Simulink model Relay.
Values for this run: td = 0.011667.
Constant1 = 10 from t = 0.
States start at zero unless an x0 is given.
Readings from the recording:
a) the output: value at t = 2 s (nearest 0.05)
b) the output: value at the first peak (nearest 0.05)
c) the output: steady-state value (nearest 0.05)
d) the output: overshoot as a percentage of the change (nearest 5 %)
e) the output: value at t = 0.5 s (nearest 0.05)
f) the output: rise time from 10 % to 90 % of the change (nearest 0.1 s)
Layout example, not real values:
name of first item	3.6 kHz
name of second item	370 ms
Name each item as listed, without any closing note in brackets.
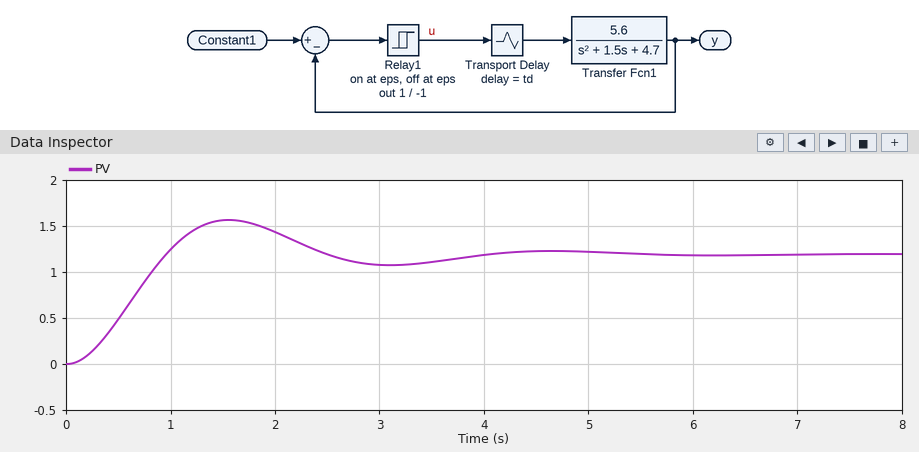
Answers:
the output: value at t = 2 s	1.45
the output: value at the first peak	1.55
the output: steady-state value	1.20
the output: overshoot as a percentage of the change	30 %
the output: value at t = 0.5 s	0.50
the output: rise time from 10 % to 90 % of the change	0.6 s
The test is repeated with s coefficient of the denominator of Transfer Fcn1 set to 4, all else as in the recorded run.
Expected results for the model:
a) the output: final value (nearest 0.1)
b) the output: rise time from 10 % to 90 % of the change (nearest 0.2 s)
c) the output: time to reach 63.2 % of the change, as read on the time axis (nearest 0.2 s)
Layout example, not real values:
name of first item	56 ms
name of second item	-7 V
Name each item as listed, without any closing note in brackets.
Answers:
the output: final value	1.2
the output: rise time from 10 % to 90 % of the change	1.4 s
the output: time to reach 63.2 % of the change, as read on the time axis	1.0 s
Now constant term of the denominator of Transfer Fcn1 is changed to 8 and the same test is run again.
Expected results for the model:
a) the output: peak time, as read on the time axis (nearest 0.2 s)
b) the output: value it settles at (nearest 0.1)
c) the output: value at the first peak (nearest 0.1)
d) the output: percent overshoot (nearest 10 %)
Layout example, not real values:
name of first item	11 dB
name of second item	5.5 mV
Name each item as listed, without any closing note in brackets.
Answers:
the output: peak time, as read on the time axis	1.2 s
the output: value it settles at	0.7
the output: value at the first peak	1.0
the output: percent overshoot	40 %
